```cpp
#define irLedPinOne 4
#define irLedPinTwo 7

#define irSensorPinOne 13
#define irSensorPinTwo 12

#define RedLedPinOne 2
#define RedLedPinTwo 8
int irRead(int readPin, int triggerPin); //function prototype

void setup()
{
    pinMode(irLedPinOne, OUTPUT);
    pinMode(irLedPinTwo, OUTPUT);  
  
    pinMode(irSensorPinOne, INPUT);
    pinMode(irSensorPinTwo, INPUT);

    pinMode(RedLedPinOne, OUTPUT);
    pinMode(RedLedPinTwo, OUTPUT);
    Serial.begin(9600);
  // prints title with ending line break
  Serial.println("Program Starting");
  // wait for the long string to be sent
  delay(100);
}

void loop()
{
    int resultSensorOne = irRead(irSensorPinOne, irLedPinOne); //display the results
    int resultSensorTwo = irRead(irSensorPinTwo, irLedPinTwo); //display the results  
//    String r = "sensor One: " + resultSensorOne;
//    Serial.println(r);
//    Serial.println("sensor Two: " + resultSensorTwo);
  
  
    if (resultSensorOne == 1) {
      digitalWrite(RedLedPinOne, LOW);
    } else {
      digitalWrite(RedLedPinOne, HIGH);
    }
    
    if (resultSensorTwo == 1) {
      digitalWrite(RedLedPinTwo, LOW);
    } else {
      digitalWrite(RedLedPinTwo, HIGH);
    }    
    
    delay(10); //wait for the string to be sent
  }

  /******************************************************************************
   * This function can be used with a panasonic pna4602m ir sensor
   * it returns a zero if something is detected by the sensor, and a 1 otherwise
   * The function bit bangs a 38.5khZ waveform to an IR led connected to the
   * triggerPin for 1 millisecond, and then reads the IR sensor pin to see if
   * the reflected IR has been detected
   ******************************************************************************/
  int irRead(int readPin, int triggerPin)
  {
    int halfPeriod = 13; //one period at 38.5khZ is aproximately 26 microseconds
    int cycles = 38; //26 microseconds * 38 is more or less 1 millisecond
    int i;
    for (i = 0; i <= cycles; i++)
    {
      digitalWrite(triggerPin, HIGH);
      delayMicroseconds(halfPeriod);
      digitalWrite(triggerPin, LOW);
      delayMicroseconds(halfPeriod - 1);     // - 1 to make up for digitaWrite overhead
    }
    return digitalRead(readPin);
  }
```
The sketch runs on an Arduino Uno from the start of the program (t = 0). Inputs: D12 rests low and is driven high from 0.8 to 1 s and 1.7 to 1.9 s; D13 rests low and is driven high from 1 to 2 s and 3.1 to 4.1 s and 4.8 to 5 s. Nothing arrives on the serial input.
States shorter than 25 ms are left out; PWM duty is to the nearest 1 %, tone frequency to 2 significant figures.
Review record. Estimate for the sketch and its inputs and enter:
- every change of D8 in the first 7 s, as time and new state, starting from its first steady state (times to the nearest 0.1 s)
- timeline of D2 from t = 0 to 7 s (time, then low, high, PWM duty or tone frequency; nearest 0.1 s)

0 s low; 0.1 s high; 0.8 s low; 1 s high; 1.7 s low; 1.9 s high
0 s low; 0.1 s high; 1 s low; 2 s high; 3.1 s low; 4.1 s high; 4.8 s low; 5 s high
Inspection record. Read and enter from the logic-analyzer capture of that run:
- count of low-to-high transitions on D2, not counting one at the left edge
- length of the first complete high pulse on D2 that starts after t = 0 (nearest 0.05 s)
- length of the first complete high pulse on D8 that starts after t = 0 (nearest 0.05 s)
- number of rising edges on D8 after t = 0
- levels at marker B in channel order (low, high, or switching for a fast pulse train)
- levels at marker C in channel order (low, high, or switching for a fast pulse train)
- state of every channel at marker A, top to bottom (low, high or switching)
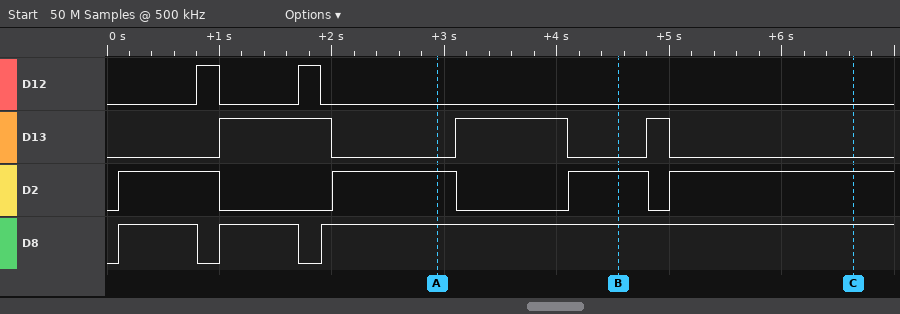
4
0.90 s
0.70 s
3
D12 low, D13 low, D2 high, D8 high
D12 low, D13 low, D2 high, D8 high
D12 low, D13 low, D2 high, D8 high
